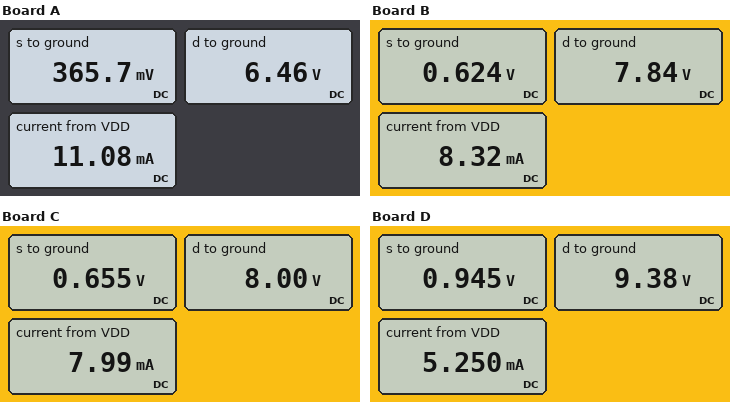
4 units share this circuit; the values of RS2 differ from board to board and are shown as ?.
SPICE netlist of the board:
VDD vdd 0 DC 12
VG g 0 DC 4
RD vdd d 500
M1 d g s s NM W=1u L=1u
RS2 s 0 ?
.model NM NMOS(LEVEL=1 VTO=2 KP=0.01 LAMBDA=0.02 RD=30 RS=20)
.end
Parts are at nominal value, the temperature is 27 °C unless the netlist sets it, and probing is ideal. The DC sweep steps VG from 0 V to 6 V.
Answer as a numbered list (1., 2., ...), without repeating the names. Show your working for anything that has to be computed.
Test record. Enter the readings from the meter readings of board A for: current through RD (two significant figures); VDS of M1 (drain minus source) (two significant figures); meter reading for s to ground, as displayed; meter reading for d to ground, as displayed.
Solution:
1. (12 V - 6.46 V) / 500 Ω = 11 mA
2. 6.46 V - 365.7 mV = 6.1 V
3. 365.7 mV
4. 6.46 V
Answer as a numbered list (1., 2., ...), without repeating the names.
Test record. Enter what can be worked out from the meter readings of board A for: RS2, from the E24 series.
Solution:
1. 33 Ω
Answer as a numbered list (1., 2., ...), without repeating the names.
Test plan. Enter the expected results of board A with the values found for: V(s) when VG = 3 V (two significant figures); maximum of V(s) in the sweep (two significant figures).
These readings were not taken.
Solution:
1. 130 mV
2. 640 mV
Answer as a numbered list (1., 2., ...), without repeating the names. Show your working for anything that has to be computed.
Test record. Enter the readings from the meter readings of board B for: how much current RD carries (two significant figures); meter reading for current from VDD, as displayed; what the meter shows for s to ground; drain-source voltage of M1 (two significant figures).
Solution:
1. (12 V - 7.84 V) / 500 Ω = 8.3 mA
2. 8.32 mA
3. 0.624 V
4. 7.84 V - 624 mV = 7.2 V
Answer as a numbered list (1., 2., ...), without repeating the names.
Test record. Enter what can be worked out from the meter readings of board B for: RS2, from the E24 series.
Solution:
1. 75 Ω
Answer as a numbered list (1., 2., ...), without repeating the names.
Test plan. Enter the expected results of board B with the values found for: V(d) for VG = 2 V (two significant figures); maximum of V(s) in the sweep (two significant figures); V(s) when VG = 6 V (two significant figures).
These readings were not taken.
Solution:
1. 12 V
2. 1.3 V
3. 1.3 V
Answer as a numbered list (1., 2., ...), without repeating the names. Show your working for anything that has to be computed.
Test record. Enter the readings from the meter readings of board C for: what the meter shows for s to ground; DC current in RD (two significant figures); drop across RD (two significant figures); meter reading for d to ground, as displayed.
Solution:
1. 0.655 V
2. (12 V - 8 V) / 500 Ω = 8.0 mA
3. 12 V - 8 V = 4.0 V
4. 8.00 V
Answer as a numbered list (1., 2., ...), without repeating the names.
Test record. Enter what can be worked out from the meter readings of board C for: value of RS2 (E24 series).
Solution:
1. 82 Ω
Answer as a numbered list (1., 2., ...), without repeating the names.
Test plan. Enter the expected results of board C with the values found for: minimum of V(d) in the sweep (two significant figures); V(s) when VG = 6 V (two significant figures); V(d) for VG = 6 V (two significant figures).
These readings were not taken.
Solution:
1. 3.3 V
2. 1.4 V
3. 3.3 V
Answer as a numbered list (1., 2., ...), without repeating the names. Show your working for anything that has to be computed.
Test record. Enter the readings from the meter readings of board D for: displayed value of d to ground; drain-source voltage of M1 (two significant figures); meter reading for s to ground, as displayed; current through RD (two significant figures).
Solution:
1. 9.38 V
2. 9.38 V - 945 mV = 8.4 V
3. 0.945 V
4. (12 V - 9.38 V) / 500 Ω = 5.2 mA
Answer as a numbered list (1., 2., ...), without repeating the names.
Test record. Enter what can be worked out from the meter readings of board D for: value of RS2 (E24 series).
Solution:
1. 180 Ω
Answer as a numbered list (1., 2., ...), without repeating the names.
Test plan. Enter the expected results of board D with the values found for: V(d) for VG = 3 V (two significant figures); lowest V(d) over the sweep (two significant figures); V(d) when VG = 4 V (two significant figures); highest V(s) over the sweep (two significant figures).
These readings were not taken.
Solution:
1. 11 V
2. 5.8 V
3. 9.4 V
4. 2.2 V
